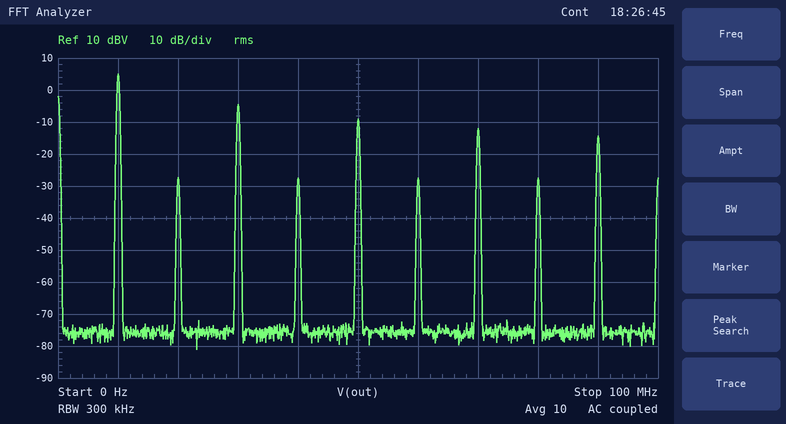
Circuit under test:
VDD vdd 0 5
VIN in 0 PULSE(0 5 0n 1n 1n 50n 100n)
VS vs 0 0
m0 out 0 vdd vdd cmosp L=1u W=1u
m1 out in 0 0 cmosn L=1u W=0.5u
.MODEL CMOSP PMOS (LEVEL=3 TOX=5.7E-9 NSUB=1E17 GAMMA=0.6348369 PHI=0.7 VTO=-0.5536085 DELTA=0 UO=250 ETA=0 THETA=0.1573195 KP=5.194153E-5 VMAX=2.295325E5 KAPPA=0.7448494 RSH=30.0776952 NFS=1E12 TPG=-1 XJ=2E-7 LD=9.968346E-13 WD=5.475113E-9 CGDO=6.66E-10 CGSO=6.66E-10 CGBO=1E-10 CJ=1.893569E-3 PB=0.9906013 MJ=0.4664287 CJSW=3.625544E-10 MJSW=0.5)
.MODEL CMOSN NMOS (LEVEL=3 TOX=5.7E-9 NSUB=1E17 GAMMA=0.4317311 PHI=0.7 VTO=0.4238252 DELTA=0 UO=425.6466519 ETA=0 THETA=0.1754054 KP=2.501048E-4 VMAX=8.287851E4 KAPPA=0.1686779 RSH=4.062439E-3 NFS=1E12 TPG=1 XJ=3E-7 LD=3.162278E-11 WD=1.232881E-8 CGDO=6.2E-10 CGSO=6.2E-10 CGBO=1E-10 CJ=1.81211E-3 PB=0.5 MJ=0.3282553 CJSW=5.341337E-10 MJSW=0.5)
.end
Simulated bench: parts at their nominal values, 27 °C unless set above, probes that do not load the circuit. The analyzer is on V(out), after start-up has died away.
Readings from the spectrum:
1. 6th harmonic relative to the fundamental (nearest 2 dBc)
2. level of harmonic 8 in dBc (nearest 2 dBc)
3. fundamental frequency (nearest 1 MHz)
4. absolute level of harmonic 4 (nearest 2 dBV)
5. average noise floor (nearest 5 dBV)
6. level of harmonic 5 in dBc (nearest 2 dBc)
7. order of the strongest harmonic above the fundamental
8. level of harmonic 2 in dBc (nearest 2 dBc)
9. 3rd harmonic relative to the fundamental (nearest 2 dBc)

-32 dBc
-32 dBc
10 MHz
-28 dBV
-75 dBV
-14 dBc
3
-32 dBc
-10 dBc
